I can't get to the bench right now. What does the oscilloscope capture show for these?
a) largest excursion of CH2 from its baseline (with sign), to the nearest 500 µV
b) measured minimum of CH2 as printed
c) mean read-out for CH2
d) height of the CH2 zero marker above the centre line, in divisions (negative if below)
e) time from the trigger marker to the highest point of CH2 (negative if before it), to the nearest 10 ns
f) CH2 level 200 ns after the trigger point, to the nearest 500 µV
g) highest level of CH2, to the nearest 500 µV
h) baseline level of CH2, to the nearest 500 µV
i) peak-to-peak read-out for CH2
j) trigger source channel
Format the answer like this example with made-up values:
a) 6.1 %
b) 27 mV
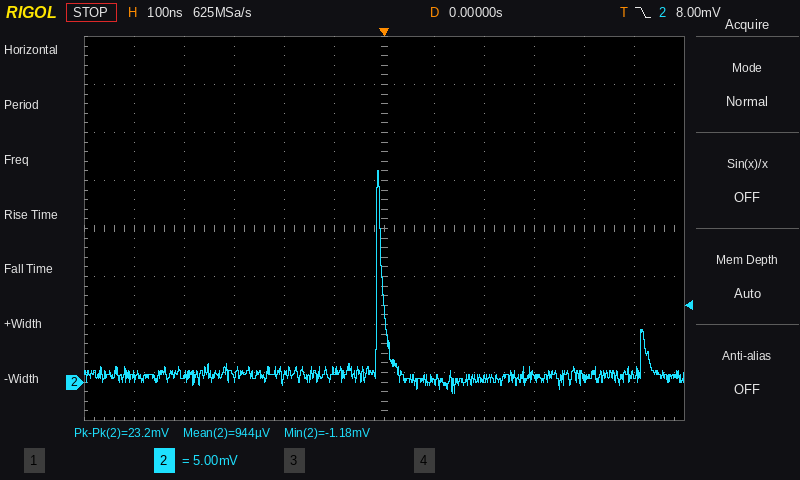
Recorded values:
a) +21.5 mV
b) -1.18 mV
c) 944 µV
d) -3.2 div
e) -10 ns
f) 500 µV
g) 22.0 mV
h) 500 µV
i) 23.2 mV
j) CH2
